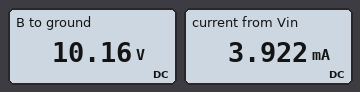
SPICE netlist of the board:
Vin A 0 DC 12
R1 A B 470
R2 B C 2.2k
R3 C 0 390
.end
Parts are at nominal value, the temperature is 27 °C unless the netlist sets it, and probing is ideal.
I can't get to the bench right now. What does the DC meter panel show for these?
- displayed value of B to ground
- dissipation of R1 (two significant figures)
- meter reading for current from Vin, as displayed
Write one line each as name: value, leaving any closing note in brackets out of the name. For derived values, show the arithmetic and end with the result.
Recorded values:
displayed value of B to ground: 10.16 V
dissipation of R1: (12 V - 10.16 V)^2 / 470 Ω = 7.2 mW
meter reading for current from Vin, as displayed: 3.922 mA
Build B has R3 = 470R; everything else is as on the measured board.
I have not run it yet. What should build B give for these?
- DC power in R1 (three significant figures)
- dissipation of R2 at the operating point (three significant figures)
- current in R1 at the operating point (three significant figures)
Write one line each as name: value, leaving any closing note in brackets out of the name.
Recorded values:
DC power in R1: 6.86 mW
dissipation of R2 at the operating point: 32.1 mW
current in R1 at the operating point: 3.82 mA
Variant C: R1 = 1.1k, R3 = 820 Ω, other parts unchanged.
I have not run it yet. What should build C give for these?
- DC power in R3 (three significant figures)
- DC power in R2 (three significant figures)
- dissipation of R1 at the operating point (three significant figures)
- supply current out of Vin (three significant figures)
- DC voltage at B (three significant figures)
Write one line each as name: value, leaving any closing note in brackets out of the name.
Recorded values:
DC power in R3: 6.96 mW
DC power in R2: 18.7 mW
dissipation of R1 at the operating point: 9.33 mW
supply current out of Vin: 2.91 mA
DC voltage at B: 8.80 V
